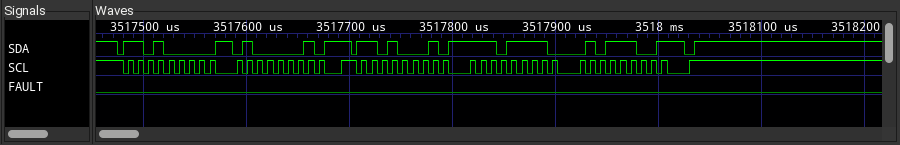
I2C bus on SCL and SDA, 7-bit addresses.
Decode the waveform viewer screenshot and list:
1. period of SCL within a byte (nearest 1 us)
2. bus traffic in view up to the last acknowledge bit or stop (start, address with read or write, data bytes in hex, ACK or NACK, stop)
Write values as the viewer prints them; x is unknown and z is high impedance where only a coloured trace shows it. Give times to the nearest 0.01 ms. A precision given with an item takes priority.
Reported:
10 us
start, address 68 write ACK, 41 ACK, repeated start, address 68 read ACK, EF ACK, 5C NACK, stop
